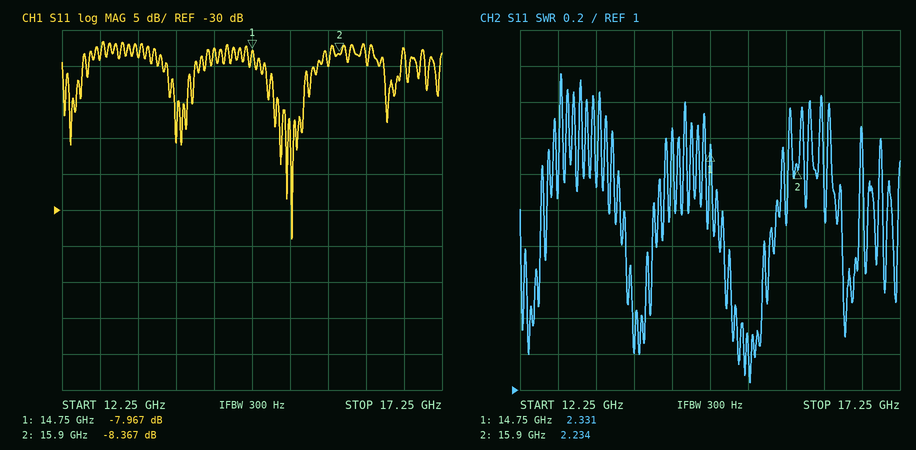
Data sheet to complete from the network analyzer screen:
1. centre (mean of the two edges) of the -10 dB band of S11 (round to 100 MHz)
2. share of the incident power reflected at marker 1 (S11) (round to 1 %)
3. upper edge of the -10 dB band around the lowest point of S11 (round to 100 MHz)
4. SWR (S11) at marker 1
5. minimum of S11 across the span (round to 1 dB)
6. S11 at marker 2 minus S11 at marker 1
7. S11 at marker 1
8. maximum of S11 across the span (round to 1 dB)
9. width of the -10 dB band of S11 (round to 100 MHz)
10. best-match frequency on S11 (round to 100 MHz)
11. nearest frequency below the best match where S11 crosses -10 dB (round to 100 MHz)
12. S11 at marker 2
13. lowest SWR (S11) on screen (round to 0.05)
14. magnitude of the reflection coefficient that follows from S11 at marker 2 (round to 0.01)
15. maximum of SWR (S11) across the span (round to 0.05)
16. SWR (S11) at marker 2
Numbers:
15.3 GHz
16 %
15.6 GHz
2.331
-34 dB
-0.400 dB
-7.967 dB
-7 dB
700 MHz
15.3 GHz
14.9 GHz
-8.367 dB
1.05
0.38
2.75
2.234
